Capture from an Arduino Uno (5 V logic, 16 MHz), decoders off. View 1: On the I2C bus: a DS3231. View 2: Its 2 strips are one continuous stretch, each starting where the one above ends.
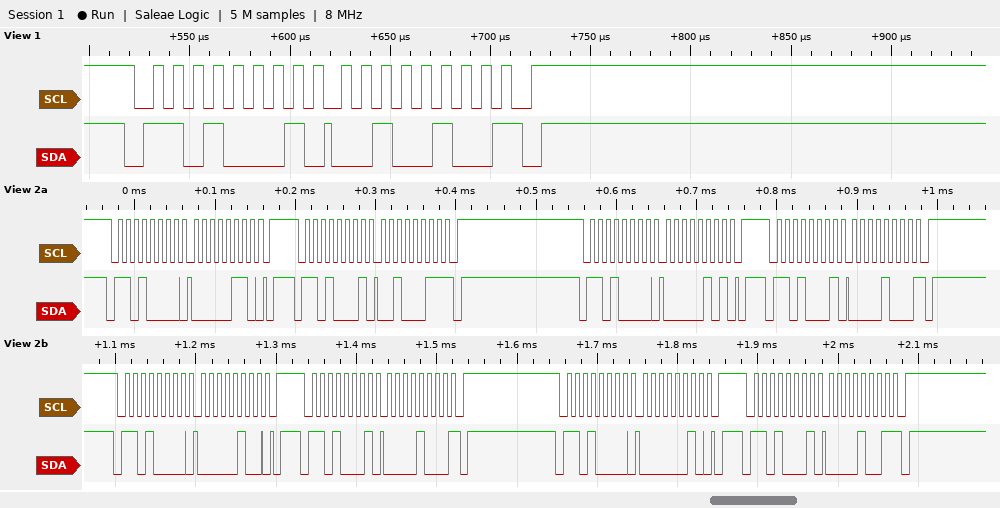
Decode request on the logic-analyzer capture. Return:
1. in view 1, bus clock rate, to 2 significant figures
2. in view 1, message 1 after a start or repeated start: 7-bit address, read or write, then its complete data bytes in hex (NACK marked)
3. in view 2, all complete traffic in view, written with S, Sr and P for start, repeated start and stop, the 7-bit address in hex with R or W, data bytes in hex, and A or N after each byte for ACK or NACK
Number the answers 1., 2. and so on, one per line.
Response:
1. 100 kHz
2. 0x68 read: 24 NACK
3. S 68W A 06 A P S 68R A 23 N P S 68W A 05 A P S 68R A 08 N P S 68W A 04 A P S 68R A 08 N P S 68W A 02 A P S 68R A 09 N P
